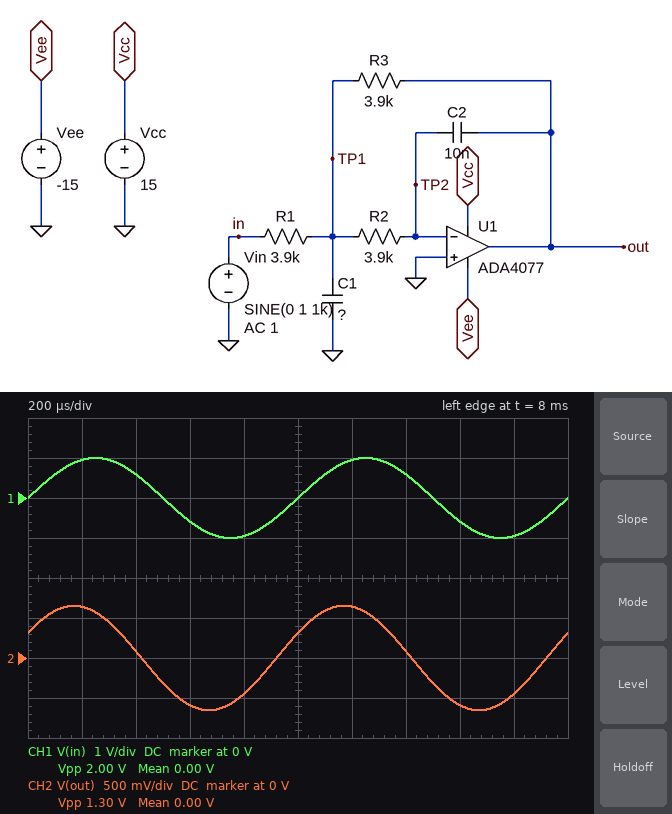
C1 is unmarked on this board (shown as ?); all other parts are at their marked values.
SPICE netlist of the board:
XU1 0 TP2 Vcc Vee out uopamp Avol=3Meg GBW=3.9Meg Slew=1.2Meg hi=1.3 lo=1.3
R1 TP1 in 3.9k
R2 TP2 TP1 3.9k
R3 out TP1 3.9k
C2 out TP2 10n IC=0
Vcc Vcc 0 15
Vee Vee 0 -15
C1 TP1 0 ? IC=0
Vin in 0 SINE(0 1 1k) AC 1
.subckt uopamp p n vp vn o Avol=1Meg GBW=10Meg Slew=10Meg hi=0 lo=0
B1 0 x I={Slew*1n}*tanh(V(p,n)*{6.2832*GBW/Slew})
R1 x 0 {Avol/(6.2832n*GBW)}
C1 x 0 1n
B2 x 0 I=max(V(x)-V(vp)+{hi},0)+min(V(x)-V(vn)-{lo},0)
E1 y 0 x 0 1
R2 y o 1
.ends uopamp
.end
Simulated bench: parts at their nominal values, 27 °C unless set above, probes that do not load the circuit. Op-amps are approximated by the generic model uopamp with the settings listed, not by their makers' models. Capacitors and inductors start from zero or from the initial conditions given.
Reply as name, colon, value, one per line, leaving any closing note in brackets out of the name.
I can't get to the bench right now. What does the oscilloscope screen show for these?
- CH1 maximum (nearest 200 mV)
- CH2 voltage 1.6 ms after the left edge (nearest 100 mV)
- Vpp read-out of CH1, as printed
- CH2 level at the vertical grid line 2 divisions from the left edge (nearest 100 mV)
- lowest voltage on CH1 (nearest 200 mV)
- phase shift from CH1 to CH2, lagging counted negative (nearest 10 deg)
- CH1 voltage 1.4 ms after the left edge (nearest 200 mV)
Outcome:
CH1 maximum: 1.0 V
CH2 voltage 1.6 ms after the left edge: -600 mV
Vpp read-out of CH1, as printed: 2.00 V
CH2 level at the vertical grid line 2 divisions from the left edge: 100 mV
lowest voltage on CH1: -1.0 V
phase shift from CH1 to CH2, lagging counted negative: 30 deg
CH1 voltage 1.4 ms after the left edge: 600 mV
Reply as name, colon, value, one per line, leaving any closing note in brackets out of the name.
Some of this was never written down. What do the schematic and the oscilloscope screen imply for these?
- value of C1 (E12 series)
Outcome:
value of C1: 390 nF
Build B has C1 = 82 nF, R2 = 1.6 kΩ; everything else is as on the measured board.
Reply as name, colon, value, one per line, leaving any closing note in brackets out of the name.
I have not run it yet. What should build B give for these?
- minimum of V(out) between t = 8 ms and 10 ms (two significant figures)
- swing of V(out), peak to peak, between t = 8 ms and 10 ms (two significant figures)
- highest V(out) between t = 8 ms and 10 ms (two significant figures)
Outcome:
minimum of V(out) between t = 8 ms and 10 ms: -1.1 V
swing of V(out), peak to peak, between t = 8 ms and 10 ms: 2.2 V
highest V(out) between t = 8 ms and 10 ms: 1.1 V
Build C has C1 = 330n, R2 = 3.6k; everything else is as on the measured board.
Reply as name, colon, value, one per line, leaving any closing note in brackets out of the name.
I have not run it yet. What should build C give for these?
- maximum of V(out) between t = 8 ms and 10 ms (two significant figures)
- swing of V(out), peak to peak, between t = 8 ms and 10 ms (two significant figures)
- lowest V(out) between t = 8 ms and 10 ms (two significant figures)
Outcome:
maximum of V(out) between t = 8 ms and 10 ms: 920 mV
swing of V(out), peak to peak, between t = 8 ms and 10 ms: 1.8 V
lowest V(out) between t = 8 ms and 10 ms: -920 mV
